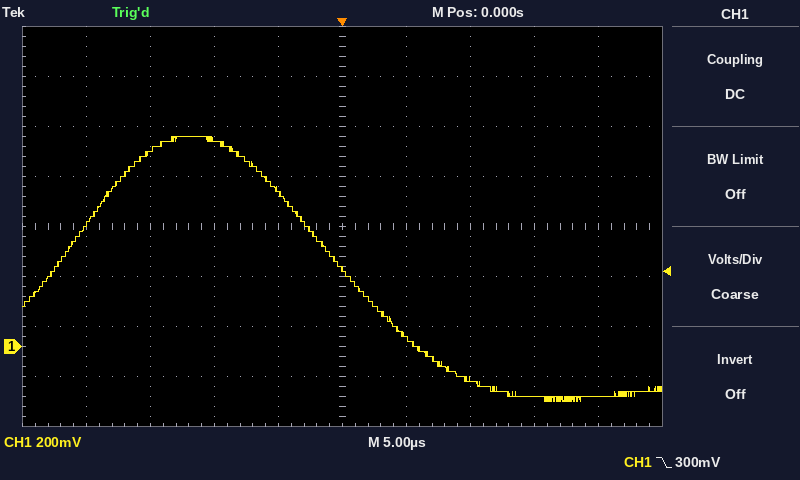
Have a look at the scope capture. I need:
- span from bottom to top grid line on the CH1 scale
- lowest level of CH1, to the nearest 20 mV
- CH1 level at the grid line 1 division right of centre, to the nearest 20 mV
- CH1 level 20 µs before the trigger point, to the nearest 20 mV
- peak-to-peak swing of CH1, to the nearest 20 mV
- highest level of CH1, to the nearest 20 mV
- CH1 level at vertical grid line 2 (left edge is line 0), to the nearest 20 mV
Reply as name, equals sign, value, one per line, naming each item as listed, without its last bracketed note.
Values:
span from bottom to top grid line on the CH1 scale = 1.6 V
lowest level of CH1, to the nearest 20 mV = -220 mV
CH1 level at the grid line 1 division right of centre, to the nearest 20 mV = 40 mV
CH1 level 20 µs before the trigger point, to the nearest 20 mV = 480 mV
peak-to-peak swing of CH1, to the nearest 20 mV = 1.06 V
highest level of CH1, to the nearest 20 mV = 840 mV
CH1 level at vertical grid line 2 (left edge is line 0), to the nearest 20 mV = 780 mV
